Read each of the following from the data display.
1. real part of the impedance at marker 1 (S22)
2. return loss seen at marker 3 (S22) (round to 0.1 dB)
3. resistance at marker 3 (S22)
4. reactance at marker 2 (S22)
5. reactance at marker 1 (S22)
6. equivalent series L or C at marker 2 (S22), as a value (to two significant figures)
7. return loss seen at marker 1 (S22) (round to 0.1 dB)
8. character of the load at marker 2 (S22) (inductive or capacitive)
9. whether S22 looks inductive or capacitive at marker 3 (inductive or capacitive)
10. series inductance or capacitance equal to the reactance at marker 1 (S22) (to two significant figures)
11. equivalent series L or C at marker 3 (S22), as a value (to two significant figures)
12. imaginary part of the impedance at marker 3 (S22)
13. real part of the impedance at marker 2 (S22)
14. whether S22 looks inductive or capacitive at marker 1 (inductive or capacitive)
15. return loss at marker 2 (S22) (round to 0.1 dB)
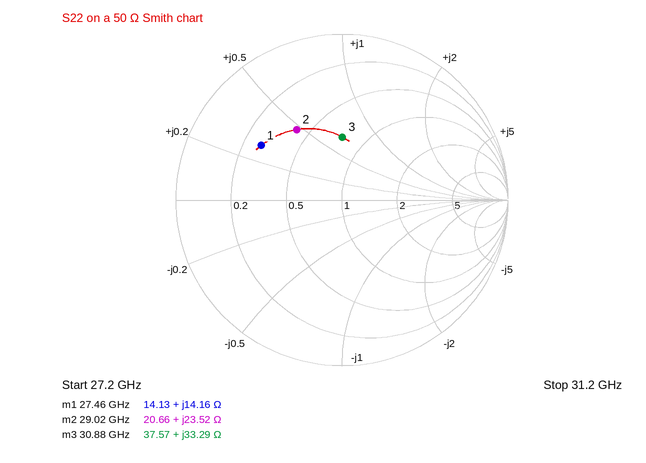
14.13 Ω
8.4 dB
37.57 Ω
+23.52 Ω
+14.16 Ω
130 pH
4.6 dB
inductive
inductive
82 pH
170 pH
+33.29 Ω
20.66 Ω
inductive
5.9 dB
